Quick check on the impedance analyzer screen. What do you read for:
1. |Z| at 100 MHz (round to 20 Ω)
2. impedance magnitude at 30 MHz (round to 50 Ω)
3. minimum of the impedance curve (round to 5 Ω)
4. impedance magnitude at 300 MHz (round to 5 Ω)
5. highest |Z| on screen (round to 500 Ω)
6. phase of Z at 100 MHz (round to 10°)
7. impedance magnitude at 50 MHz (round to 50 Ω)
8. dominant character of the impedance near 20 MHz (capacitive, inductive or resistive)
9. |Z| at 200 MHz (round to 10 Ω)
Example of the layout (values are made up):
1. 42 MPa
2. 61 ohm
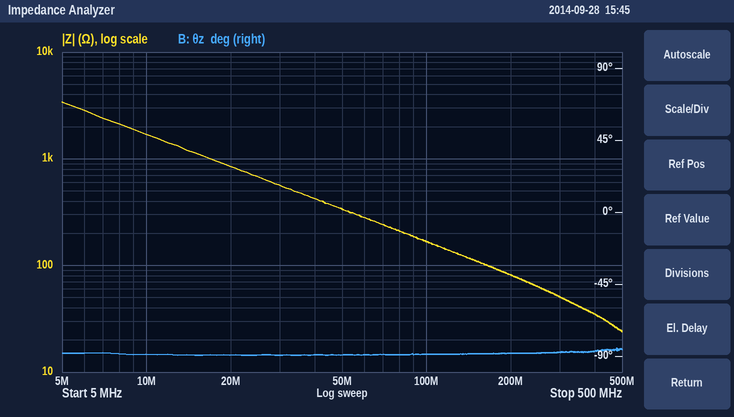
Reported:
1. 160 Ω
2. 550 Ω
3. 25 Ω
4. 50 Ω
5. 3.5 kΩ
6. -90°
7. 350 Ω
8. capacitive
9. 80 Ω
